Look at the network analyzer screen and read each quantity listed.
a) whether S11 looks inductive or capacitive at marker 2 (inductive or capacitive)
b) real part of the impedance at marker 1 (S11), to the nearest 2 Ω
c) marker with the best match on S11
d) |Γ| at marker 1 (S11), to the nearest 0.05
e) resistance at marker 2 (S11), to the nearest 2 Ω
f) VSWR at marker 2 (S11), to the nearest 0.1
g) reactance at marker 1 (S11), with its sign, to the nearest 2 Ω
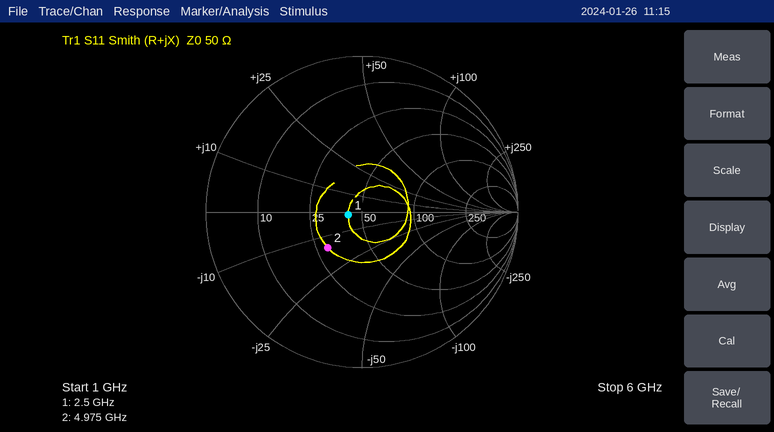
capacitive
42 Ω
marker 1
0.10
30 Ω
1.9
-2 Ω
